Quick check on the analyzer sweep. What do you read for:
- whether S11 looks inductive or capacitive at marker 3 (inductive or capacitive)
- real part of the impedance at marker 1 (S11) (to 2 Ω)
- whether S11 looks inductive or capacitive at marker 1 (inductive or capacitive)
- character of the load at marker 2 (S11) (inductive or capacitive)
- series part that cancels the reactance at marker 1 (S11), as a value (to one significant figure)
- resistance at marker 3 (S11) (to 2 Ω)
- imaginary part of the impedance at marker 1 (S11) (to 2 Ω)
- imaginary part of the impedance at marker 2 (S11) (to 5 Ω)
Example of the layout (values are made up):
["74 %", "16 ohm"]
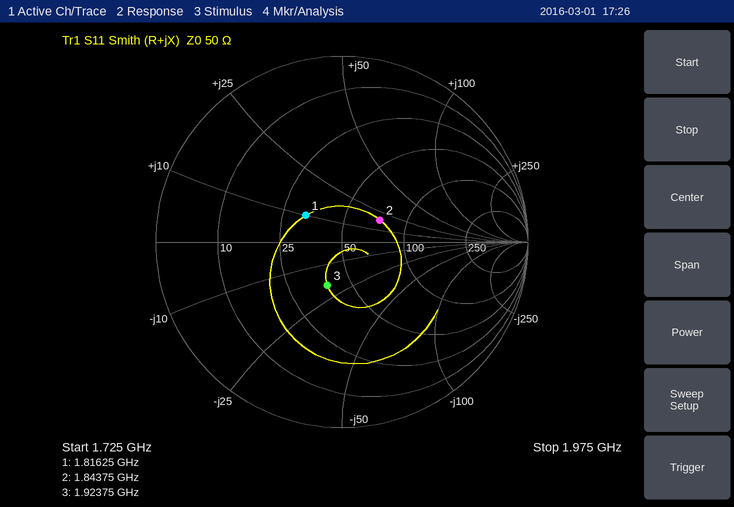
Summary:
["capacitive", "32 Ω", "inductive", "inductive", "9 pF", "38 Ω", "+10 Ω", "+20 Ω"]
